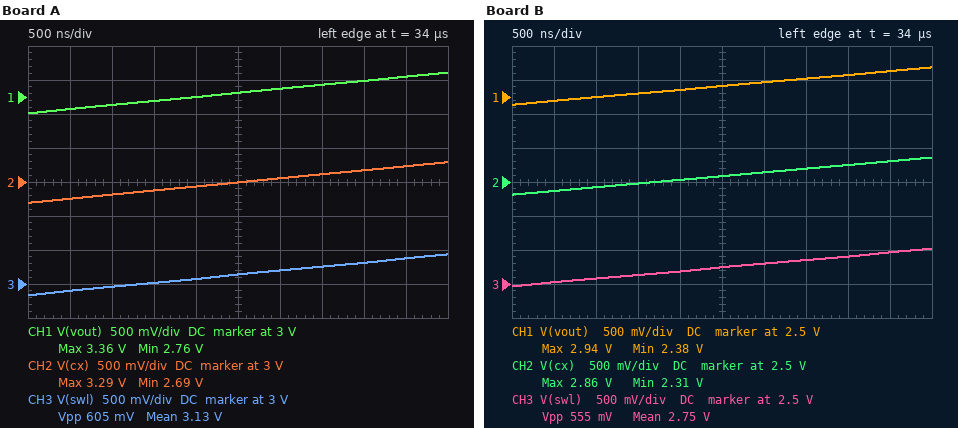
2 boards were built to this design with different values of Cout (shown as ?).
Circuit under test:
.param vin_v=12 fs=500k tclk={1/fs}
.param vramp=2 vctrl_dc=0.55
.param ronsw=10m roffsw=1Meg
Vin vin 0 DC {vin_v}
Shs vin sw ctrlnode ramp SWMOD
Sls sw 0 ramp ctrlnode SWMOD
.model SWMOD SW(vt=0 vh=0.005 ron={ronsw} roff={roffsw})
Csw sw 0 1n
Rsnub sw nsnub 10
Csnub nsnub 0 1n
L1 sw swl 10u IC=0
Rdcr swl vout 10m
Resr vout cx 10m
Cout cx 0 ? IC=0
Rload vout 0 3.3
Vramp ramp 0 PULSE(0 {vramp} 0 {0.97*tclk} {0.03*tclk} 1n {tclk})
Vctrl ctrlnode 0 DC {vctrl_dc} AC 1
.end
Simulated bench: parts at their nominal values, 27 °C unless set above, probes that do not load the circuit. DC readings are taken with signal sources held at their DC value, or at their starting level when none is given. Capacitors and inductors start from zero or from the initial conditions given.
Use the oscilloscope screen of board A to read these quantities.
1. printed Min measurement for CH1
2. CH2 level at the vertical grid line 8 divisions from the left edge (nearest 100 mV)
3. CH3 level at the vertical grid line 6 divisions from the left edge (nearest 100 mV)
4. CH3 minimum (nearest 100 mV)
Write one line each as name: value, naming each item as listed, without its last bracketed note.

printed Min measurement for CH1: 2.76 V
CH2 level at the vertical grid line 8 divisions from the left edge: 3.2 V
CH3 level at the vertical grid line 6 divisions from the left edge: 3.2 V
CH3 minimum: 2.8 V
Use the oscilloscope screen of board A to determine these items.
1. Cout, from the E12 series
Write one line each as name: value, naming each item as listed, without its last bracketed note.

Cout, from the E12 series: 56 µF
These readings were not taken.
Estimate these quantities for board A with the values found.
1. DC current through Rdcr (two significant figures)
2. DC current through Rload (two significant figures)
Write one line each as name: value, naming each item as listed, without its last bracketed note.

DC current through Rdcr: 3.6 A
DC current through Rload: 3.6 A
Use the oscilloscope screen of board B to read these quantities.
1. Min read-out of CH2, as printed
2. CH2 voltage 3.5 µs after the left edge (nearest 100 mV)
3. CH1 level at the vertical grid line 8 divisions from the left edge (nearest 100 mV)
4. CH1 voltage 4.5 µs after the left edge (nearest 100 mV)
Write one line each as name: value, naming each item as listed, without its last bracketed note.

Min read-out of CH2, as printed: 2.31 V
CH2 voltage 3.5 µs after the left edge: 2.7 V
CH1 level at the vertical grid line 8 divisions from the left edge: 2.8 V
CH1 voltage 4.5 µs after the left edge: 2.9 V
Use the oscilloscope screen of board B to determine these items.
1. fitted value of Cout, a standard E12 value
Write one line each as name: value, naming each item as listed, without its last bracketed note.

fitted value of Cout, a standard E12 value: 68 µF
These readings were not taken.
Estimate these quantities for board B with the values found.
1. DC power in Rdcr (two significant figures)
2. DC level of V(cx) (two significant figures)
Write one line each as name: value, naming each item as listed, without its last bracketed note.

DC power in Rdcr: 130 mW
DC level of V(cx): 12 V
